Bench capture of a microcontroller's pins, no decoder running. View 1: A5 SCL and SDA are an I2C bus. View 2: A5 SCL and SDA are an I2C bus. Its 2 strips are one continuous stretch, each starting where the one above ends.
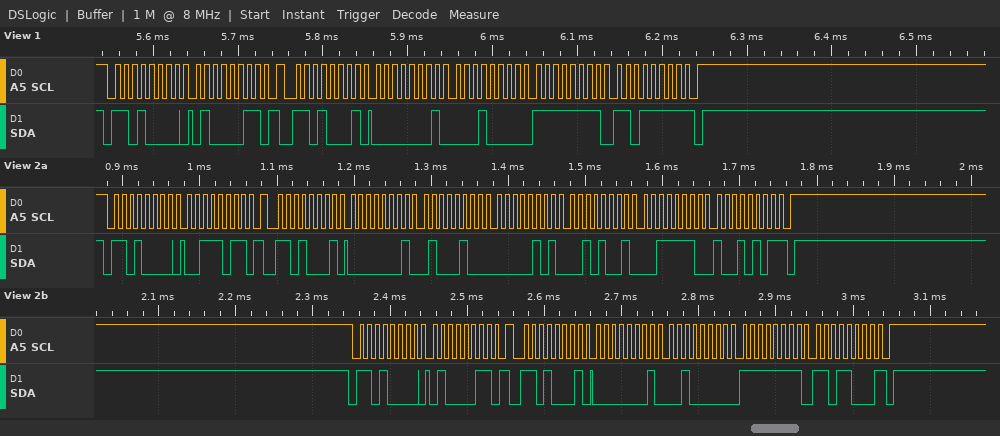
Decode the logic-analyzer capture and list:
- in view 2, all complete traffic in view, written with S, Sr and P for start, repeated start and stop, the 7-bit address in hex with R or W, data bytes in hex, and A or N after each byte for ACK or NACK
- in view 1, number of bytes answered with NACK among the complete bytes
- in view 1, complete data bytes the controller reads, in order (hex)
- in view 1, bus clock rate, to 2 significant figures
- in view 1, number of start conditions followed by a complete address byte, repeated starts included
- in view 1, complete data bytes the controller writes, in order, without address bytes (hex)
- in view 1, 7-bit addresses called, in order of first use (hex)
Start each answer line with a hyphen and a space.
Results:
- S 68W A 3B A Sr 68R A 01 A 44 A 05 A 29 A 3E A 95 N P S 68W A 43 A Sr 68R A 01 A 20 A FF A D8 N P
- 1
- 01 10 FF DF
- 100 kHz
- 2
- 43
- 0x68
